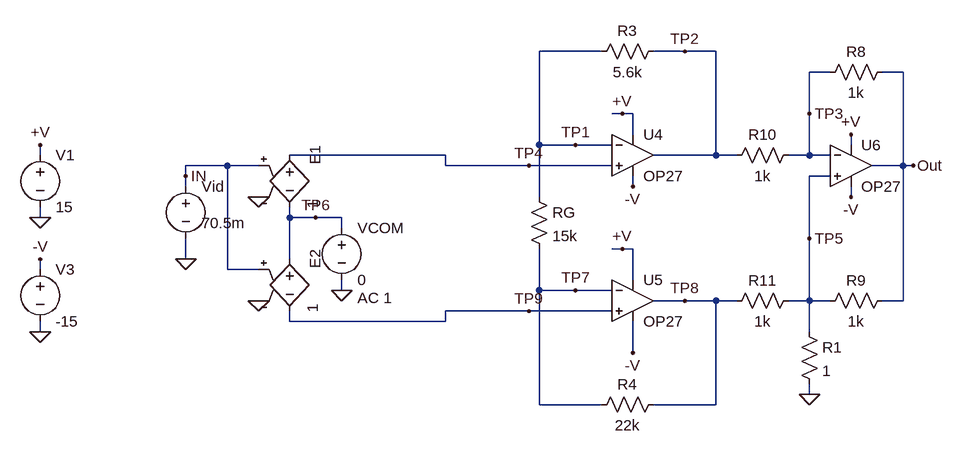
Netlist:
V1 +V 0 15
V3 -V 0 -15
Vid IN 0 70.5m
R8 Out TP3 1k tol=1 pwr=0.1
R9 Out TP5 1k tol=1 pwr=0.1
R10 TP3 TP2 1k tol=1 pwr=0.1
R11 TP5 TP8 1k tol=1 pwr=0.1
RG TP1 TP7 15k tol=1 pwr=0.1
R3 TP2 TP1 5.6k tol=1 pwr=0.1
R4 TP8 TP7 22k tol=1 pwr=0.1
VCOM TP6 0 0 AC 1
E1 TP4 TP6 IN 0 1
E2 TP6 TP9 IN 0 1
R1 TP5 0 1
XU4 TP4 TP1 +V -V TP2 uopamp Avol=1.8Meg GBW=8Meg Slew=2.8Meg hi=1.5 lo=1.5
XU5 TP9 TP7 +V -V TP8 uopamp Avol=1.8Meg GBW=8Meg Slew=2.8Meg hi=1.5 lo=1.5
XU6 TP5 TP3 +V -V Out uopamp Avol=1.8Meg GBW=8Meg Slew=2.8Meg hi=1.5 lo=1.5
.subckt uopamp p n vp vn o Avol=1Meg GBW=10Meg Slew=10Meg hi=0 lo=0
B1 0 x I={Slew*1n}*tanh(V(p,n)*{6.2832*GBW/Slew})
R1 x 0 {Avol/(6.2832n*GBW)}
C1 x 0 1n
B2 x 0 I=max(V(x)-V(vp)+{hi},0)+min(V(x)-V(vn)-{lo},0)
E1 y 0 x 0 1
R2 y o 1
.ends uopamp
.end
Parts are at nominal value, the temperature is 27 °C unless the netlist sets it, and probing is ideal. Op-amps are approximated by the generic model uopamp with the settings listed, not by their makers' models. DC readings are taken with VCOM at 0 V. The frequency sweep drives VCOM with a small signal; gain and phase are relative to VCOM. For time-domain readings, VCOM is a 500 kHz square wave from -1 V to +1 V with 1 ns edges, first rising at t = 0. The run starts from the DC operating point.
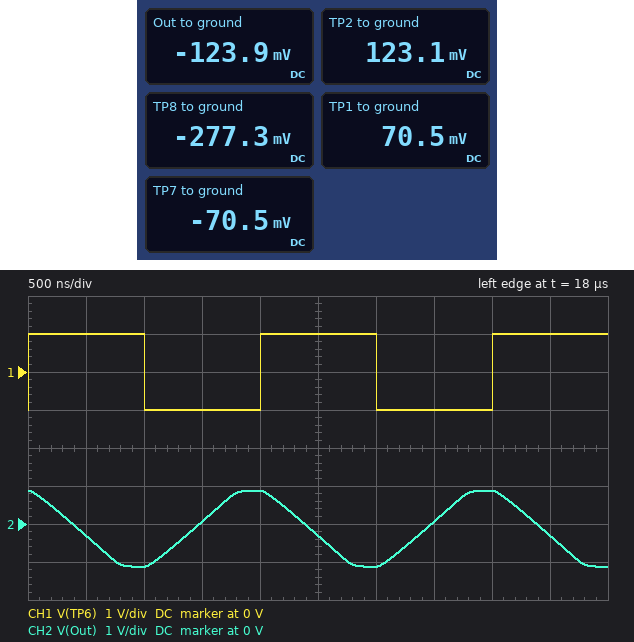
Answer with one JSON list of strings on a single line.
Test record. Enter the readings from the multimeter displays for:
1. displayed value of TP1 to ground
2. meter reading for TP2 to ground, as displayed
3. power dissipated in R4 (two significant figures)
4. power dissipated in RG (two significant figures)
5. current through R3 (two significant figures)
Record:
["70.5 mV", "123.1 mV", "1.9 µW", "1.3 µW", "9.4 µA"]
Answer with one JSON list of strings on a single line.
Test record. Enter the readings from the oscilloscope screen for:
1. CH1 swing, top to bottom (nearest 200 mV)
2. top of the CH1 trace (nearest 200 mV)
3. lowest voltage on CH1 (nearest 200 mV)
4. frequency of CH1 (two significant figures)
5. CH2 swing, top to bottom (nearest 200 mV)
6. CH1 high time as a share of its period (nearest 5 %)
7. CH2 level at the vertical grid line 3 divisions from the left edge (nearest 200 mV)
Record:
["2.0 V", "1.0 V", "-1.0 V", "500 kHz", "2.0 V", "50 %", "0 V"]
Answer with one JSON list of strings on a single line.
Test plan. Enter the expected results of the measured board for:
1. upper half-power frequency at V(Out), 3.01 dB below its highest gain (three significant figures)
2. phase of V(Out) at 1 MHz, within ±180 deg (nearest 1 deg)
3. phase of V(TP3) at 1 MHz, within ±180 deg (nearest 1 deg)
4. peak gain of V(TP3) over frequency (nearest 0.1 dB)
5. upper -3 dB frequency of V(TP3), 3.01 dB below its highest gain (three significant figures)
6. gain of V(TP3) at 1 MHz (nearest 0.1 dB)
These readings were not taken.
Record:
["3.34 MHz", "159 deg", "69 deg", "-9.5 dB", "14.2 MHz", "-18.4 dB"]
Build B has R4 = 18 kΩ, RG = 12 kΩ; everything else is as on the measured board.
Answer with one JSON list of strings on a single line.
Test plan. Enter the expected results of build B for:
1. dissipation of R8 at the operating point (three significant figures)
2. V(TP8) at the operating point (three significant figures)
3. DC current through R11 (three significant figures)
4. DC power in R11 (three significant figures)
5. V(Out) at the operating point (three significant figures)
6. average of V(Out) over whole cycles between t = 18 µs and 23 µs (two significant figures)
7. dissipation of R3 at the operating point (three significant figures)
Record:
["18.7 µW", "-282 mV", "282 µA", "79.3 µW", "-137 mV", "-140 mV", "773 nW"]
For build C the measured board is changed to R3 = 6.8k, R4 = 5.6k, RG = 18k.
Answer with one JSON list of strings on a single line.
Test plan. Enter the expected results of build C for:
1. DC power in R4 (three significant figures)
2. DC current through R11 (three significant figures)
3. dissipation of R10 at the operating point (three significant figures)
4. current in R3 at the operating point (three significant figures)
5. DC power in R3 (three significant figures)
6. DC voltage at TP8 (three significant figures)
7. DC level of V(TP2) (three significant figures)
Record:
["344 nW", "114 µA", "15.4 µW", "7.83 µA", "417 nW", "-114 mV", "124 mV"]
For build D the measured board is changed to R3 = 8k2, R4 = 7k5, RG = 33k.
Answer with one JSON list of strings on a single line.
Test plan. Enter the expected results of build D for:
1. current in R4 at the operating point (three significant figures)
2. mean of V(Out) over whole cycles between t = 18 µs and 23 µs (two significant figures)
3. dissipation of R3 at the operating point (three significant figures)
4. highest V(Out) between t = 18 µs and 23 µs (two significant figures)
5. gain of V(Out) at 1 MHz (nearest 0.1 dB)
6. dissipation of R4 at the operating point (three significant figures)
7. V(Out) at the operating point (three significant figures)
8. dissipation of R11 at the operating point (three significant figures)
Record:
["4.27 µA", "-110 mV", "150 nW", "890 mV", "-0.3 dB", "137 nW", "-106 mV", "10.5 µW"]
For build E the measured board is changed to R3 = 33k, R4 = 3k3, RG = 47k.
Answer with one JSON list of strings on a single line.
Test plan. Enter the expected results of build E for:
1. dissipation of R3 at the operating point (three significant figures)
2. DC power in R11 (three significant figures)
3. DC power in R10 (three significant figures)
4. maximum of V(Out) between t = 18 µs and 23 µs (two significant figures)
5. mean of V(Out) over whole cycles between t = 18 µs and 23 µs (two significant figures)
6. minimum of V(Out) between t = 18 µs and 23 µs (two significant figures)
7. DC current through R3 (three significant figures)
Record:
["297 nW", "6.42 µW", "28.8 µW", "830 mV", "-170 mV", "-1.2 V", "3.00 µA"]
